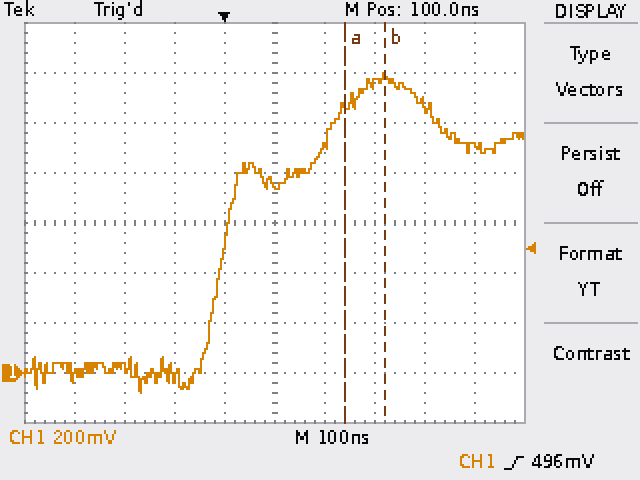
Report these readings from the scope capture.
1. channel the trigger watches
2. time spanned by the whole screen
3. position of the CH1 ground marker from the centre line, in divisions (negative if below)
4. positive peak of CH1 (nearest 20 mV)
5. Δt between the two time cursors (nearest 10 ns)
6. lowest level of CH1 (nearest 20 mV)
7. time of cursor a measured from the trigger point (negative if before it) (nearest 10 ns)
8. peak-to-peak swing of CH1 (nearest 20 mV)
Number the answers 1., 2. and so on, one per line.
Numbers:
1. CH1
2. 1 µs
3. -3.0 div
4. 1.20 V
5. 80 ns
6. -80 mV
7. +240 ns
8. 1.28 V
